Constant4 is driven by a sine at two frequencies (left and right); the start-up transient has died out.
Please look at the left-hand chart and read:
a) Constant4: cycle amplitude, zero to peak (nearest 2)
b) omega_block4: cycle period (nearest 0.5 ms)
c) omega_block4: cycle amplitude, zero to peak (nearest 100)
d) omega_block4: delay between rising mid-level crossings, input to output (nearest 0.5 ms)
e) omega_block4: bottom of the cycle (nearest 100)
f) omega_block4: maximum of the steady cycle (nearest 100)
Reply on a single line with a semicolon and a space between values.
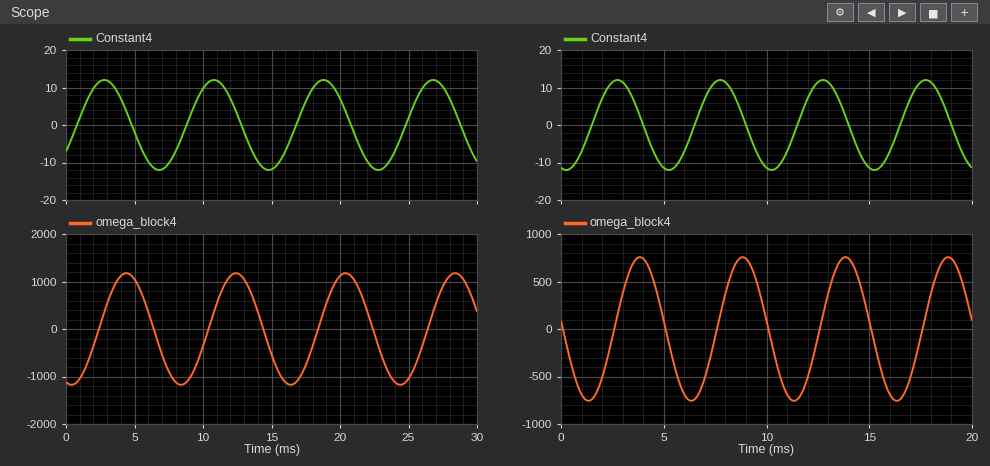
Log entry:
12; 8.0 ms; 1200; 1.5 ms; -1200; 1200
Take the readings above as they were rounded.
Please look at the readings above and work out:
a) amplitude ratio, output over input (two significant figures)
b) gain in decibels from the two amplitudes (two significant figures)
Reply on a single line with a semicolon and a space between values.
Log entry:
100; 40 dB
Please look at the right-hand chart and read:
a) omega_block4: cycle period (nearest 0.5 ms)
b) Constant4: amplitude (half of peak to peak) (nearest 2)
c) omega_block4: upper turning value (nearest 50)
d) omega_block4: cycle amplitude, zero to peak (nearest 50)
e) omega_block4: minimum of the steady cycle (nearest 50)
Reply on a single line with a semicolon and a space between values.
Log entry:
5.0 ms; 12; 750; 750; -750
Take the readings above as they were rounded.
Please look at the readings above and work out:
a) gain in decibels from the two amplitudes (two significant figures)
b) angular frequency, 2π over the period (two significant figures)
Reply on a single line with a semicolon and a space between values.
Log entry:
36 dB; 1.3 rad/ms
